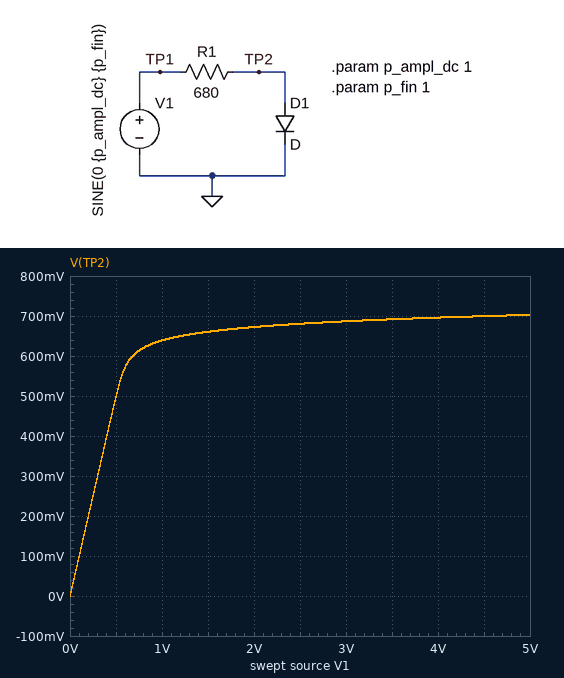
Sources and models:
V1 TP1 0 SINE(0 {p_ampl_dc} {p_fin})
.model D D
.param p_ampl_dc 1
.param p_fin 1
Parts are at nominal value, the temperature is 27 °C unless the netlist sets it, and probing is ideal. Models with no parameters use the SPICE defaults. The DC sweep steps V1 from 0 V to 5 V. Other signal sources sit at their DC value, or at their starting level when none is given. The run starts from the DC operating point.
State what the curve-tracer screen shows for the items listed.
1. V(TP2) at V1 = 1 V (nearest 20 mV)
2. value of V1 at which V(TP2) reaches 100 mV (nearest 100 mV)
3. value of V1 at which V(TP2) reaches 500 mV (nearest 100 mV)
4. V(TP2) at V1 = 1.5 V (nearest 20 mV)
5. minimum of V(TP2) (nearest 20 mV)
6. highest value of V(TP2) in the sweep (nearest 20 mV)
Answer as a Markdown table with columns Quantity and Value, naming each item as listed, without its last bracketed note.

| Quantity | Value |
|---|---|
| V(TP2) at V1 = 1 V | 640 mV |
| value of V1 at which V(TP2) reaches 100 mV | 100 mV |
| value of V1 at which V(TP2) reaches 500 mV | 500 mV |
| V(TP2) at V1 = 1.5 V | 660 mV |
| minimum of V(TP2) | 0 V |
| highest value of V(TP2) in the sweep | 700 mV |
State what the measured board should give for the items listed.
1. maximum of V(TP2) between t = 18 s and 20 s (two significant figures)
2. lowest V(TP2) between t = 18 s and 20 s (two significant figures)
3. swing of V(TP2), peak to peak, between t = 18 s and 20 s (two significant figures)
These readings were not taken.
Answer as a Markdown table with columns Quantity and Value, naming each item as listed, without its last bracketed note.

| Quantity | Value |
|---|---|
| maximum of V(TP2) between t = 18 s and 20 s | 640 mV |
| lowest V(TP2) between t = 18 s and 20 s | -1.0 V |
| swing of V(TP2), peak to peak, between t = 18 s and 20 s | 1.6 V |
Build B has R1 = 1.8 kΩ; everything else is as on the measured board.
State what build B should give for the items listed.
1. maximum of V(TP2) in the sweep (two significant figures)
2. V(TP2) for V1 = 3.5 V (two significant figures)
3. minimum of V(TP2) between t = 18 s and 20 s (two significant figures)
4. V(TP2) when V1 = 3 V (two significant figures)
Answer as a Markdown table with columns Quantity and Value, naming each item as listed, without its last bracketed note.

| Quantity | Value |
|---|---|
| maximum of V(TP2) in the sweep | 680 mV |
| V(TP2) for V1 = 3.5 V | 670 mV |
| minimum of V(TP2) between t = 18 s and 20 s | -1.0 V |
| V(TP2) when V1 = 3 V | 660 mV |
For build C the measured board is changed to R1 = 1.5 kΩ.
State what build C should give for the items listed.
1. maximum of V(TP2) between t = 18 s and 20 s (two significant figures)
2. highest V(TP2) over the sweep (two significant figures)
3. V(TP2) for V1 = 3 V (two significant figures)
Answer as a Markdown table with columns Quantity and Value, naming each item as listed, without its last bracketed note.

| Quantity | Value |
|---|---|
| maximum of V(TP2) between t = 18 s and 20 s | 620 mV |
| highest V(TP2) over the sweep | 680 mV |
| V(TP2) for V1 = 3 V | 670 mV |
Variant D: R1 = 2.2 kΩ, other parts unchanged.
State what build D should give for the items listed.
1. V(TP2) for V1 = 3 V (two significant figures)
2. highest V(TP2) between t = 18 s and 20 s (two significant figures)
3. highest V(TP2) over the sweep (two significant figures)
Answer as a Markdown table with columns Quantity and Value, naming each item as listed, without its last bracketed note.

| Quantity | Value |
|---|---|
| V(TP2) for V1 = 3 V | 660 mV |
| highest V(TP2) between t = 18 s and 20 s | 610 mV |
| highest V(TP2) over the sweep | 670 mV |
